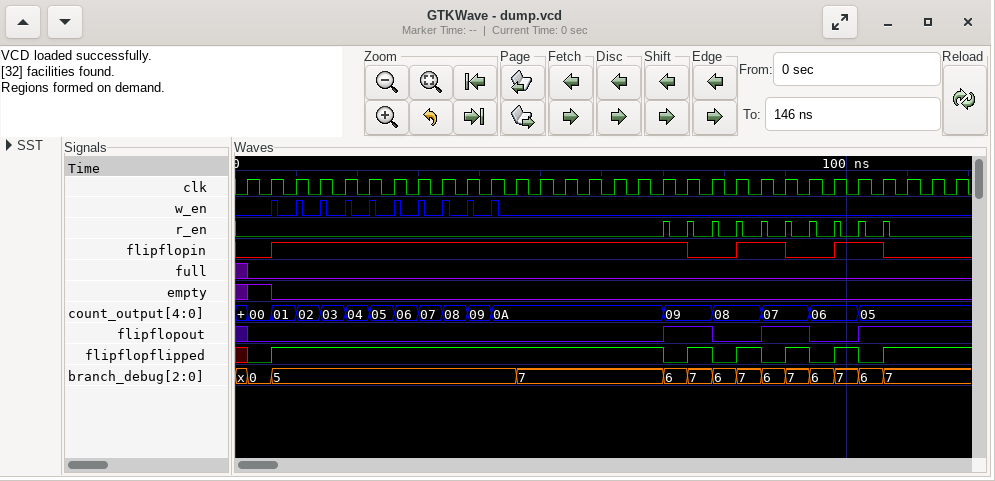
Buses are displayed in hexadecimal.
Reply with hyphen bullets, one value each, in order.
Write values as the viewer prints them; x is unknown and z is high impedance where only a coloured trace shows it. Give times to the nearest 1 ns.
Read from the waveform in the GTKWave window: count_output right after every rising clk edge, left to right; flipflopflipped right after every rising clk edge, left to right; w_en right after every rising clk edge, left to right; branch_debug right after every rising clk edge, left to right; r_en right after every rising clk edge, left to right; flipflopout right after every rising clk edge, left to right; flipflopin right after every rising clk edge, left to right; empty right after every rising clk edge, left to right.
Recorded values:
- 00, 01, 02, 03, 04, 05, 06, 07, 08, 09, 0A, 0A, 0A, 0A, 0A, 0A, 0A, 09, 09, 08, 08, 07, 07, 06, 06, 05, 05, 05, 05, 05
- 0 1 1 1 1 1 1 1 1 1 1 1 1 1 1 1 1 0 1 0 1 0 1 0 1 0 1 1 1 1
- 0 1 1 1 1 1 1 1 1 1 1 0 0 0 0 0 0 0 0 0 0 0 0 0 0 0 0 0 0 0
- 0, 5, 5, 5, 5, 5, 5, 5, 5, 5, 5, 7, 7, 7, 7, 7, 7, 6, 7, 6, 7, 6, 7, 6, 7, 6, 7, 7, 7, 7
- 0 0 0 0 0 0 0 0 0 0 0 0 0 0 0 0 0 1 1 1 1 1 1 1 1 1 1 0 0 0
- 0 0 0 0 0 0 0 0 0 0 0 0 0 0 0 0 0 1 1 0 0 1 1 0 0 1 1 1 1 1
- 0 1 1 1 1 1 1 1 1 1 1 1 1 1 1 1 1 1 0 0 1 1 0 0 1 1 0 0 0 0
- 1 0 0 0 0 0 0 0 0 0 0 0 0 0 0 0 0 0 0 0 0 0 0 0 0 0 0 0 0 0
